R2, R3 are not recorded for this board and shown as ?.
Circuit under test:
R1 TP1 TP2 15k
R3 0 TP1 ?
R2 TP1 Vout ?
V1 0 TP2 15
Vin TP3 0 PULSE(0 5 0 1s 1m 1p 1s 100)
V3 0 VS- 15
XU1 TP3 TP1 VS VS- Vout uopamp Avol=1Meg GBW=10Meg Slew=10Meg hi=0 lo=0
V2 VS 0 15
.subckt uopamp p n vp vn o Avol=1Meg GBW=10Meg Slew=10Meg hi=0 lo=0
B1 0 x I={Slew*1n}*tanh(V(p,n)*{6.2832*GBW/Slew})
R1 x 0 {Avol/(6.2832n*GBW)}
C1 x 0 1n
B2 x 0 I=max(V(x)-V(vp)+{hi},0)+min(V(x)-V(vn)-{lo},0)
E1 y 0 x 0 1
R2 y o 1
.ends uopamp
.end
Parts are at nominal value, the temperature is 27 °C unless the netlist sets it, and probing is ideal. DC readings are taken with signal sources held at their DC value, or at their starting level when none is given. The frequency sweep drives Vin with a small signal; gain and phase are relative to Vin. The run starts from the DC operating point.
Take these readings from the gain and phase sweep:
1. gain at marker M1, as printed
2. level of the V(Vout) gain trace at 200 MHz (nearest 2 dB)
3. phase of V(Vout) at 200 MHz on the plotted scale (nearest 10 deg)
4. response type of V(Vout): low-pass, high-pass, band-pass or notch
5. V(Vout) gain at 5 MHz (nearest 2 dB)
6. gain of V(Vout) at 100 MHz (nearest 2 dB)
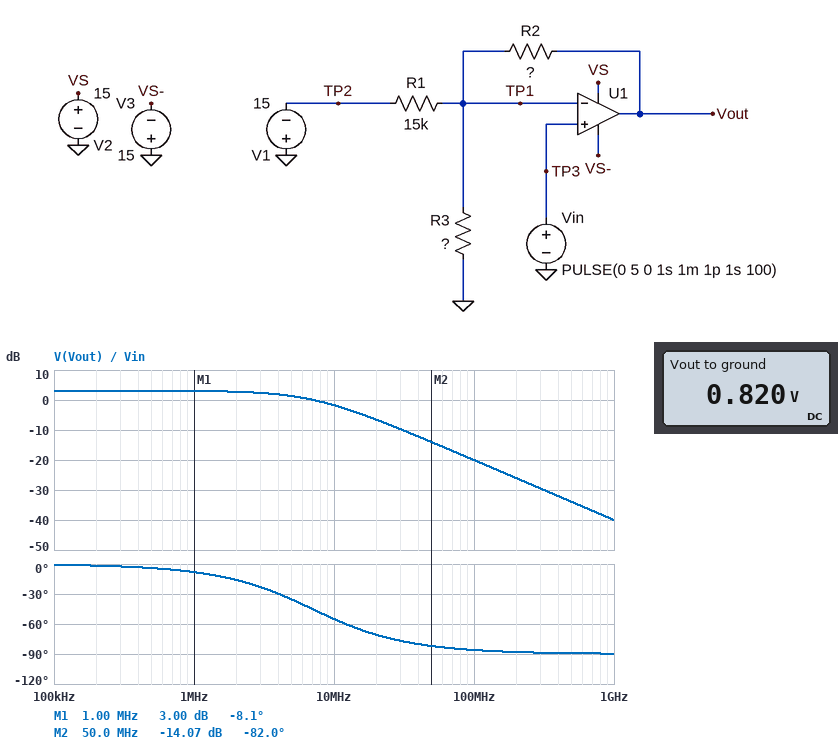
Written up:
3.00 dB
-26 dB
-90 deg
low-pass
2 dB
-20 dB
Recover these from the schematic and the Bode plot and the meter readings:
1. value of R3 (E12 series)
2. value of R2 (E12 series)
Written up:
2.2 kΩ
820 Ω
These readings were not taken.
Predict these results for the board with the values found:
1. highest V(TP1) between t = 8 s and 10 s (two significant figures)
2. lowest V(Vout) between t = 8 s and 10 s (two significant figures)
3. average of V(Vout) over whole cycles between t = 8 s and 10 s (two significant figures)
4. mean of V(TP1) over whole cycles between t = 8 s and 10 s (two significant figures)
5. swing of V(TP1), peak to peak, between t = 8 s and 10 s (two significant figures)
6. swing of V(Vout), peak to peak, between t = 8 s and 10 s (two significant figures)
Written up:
5.0 V
820 mV
4.4 V
2.5 V
5.0 V
7.1 V
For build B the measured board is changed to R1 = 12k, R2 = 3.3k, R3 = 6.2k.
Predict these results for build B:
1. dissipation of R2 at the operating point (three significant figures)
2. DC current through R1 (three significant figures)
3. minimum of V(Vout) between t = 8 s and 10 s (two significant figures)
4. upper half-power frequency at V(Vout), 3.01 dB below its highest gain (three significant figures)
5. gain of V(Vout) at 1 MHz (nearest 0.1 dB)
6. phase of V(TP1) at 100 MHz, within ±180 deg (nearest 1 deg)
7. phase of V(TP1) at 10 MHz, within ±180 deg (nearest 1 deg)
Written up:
5.16 mW
1.25 mA
4.1 V
5.53 MHz
5.0 dB
-87 deg
-61 deg
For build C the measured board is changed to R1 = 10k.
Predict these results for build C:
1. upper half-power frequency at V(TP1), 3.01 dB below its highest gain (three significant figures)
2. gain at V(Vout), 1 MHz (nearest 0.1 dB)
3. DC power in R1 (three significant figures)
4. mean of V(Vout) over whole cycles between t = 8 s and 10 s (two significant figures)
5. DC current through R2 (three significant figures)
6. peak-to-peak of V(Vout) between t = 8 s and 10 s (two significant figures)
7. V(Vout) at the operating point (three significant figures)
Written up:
6.87 MHz
3.2 dB
22.5 mW
4.9 V
1.50 mA
7.3 V
1.23 V
